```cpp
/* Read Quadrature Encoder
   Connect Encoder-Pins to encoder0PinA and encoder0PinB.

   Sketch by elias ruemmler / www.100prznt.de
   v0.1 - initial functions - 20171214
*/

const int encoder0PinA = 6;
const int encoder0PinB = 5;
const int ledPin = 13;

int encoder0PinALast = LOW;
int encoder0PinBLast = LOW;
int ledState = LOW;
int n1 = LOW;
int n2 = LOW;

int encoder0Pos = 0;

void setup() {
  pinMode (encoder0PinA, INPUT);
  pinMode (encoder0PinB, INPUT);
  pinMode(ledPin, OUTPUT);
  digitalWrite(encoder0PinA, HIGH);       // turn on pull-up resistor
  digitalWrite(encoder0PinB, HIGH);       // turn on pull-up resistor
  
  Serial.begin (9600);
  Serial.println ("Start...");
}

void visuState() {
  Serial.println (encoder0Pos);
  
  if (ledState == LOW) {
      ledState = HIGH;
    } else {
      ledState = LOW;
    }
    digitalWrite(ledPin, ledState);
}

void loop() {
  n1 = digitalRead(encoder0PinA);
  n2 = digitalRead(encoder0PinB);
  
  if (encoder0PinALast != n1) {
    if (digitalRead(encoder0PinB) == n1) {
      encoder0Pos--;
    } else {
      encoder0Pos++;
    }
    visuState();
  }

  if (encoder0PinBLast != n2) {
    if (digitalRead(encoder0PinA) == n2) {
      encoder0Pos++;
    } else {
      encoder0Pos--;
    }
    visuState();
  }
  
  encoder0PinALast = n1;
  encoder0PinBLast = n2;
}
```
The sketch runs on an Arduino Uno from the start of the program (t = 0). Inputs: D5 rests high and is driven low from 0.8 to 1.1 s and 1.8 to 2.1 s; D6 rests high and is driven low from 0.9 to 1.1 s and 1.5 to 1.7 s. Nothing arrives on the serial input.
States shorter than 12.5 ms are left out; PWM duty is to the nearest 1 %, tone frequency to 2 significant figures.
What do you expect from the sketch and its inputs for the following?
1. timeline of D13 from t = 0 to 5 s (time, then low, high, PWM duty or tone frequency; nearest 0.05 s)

0 s low; 0.8 s high; 0.9 s low; 1.5 s high; 1.7 s low; 1.8 s high; 2.1 s low
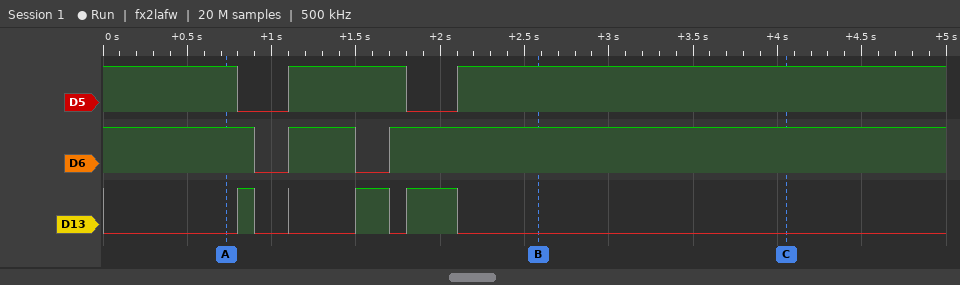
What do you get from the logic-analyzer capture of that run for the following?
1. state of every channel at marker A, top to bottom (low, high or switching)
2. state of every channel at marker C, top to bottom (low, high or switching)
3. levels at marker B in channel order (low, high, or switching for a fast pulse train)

D5 high, D6 high, D13 low
D5 high, D6 high, D13 low
D5 high, D6 high, D13 low
